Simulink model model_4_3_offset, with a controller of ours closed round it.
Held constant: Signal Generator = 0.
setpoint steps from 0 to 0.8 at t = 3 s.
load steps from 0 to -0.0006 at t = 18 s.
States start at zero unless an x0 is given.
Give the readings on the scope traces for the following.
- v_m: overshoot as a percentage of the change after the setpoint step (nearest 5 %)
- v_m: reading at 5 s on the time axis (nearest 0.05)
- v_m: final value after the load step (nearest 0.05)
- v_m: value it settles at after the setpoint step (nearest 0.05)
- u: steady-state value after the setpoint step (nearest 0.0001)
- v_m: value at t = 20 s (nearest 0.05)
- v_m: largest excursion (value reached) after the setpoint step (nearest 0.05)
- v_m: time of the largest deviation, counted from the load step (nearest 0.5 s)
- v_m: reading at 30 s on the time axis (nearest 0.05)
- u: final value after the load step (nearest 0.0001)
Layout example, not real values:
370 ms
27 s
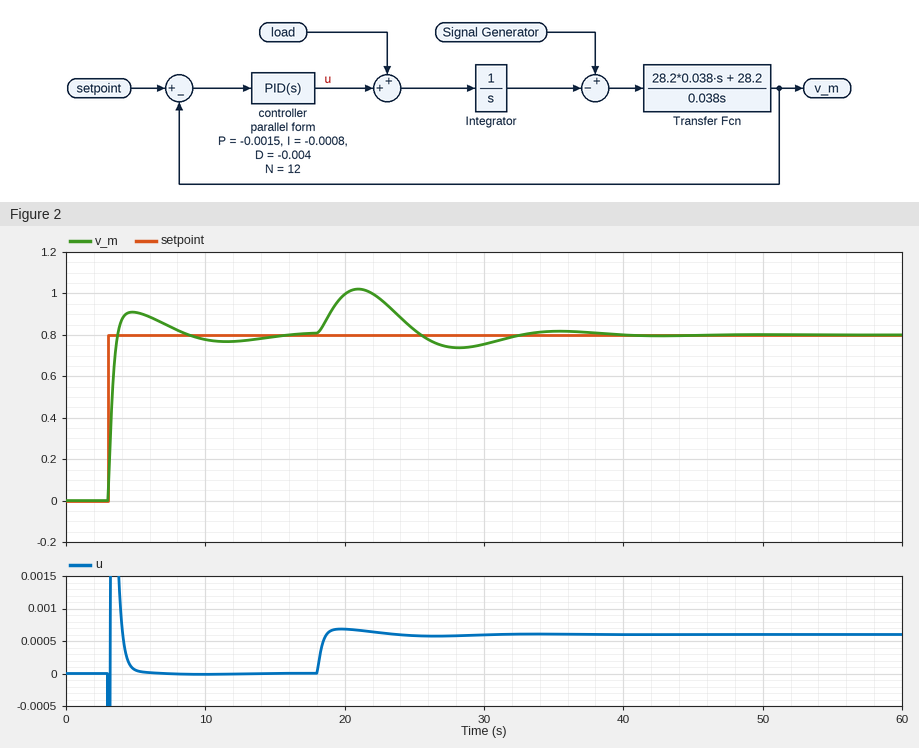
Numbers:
15 %
0.90
0.80
0.80
0.0000
1.00
0.90
3.0 s
0.75
0.0006
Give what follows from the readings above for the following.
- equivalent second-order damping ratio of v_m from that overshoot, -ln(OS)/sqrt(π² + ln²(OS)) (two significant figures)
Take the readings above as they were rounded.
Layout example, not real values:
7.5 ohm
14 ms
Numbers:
0.52
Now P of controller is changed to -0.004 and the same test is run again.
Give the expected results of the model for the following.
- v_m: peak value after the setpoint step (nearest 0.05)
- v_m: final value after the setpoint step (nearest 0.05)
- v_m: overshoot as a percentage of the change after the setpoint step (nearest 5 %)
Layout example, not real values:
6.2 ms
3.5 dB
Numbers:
0.95
0.80
20 %
